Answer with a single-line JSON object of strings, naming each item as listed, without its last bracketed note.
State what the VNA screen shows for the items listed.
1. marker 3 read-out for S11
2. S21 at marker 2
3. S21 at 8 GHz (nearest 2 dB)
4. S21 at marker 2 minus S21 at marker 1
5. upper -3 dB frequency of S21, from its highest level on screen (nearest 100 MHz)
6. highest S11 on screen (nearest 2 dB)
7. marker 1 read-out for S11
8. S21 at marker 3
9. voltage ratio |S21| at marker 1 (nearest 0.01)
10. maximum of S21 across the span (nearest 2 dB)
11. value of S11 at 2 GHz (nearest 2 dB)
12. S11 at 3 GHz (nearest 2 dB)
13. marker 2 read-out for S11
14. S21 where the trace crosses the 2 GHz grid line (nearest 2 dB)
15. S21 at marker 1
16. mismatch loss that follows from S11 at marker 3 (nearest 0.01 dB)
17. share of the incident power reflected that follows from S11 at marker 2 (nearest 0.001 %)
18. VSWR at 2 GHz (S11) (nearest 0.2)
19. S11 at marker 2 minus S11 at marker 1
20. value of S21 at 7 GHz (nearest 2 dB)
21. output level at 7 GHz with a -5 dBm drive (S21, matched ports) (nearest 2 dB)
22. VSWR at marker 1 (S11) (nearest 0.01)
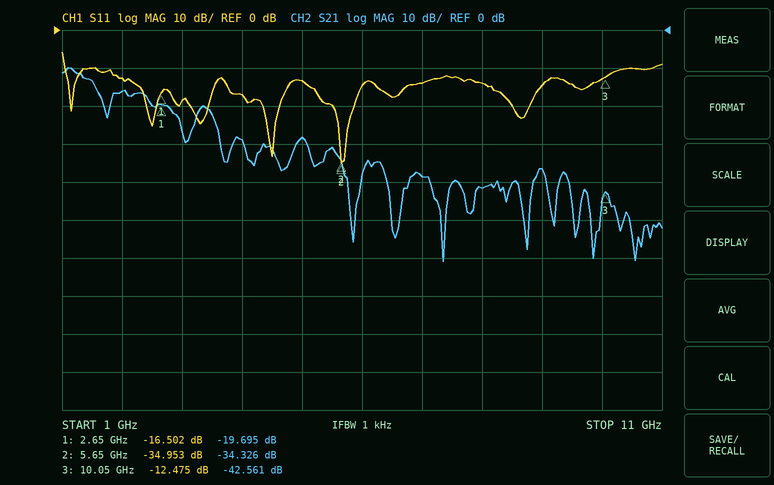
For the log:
{"marker 3 read-out for S11": "-12.475 dB", "S21 at marker 2": "-34.326 dB", "S21 at 8 GHz": "-42 dB", "S21 at marker 2 minus S21 at marker 1": "-14.631 dB", "upper -3 dB frequency of S21, from its highest level on screen": "1.4 GHz", "highest S11 on screen": "-6 dB", "marker 1 read-out for S11": "-16.502 dB", "S21 at marker 3": "-42.561 dB", "voltage ratio |S21| at marker 1": "0.10", "maximum of S21 across the span": "-10 dB", "value of S11 at 2 GHz": "-12 dB", "S11 at 3 GHz": "-18 dB", "marker 2 read-out for S11": "-34.953 dB", "S21 where the trace crosses the 2 GHz grid line": "-16 dB", "S21 at marker 1": "-19.695 dB", "mismatch loss that follows from S11 at marker 3": "0.25 dB", "share of the incident power reflected that follows from S11 at marker 2": "0.032 %", "VSWR at 2 GHz (S11)": "1.6", "S11 at marker 2 minus S11 at marker 1": "-18.451 dB", "value of S21 at 7 GHz": "-38 dB", "output level at 7 GHz with a -5 dBm drive (S21, matched ports)": "-44 dBm", "VSWR at marker 1 (S11)": "1.35"}
